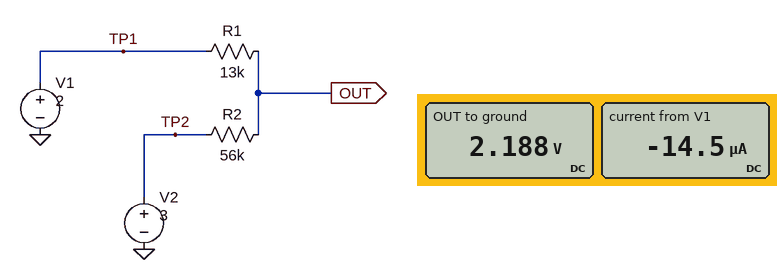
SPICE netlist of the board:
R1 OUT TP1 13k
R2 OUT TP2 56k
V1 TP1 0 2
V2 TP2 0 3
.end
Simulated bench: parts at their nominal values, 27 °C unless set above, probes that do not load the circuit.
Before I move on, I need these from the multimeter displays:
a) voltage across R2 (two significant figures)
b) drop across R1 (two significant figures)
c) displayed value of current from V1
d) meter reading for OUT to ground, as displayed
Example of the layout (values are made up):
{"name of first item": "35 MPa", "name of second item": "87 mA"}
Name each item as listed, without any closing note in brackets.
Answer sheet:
{"voltage across R2": "810 mV", "drop across R1": "190 mV", "displayed value of current from V1": "-14.5 µA", "meter reading for OUT to ground, as displayed": "2.188 V"}
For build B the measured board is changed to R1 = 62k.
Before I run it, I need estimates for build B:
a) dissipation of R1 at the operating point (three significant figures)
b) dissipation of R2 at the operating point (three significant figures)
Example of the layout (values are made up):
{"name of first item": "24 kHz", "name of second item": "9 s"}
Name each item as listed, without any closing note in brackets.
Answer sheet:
{"dissipation of R1 at the operating point": "4.45 µW", "dissipation of R2 at the operating point": "4.02 µW"}
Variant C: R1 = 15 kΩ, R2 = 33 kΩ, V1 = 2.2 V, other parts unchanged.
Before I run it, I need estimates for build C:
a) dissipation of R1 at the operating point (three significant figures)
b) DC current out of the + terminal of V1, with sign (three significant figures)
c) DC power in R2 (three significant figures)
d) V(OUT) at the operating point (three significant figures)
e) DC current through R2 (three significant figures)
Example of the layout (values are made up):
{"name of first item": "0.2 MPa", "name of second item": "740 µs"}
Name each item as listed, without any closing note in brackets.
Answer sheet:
{"dissipation of R1 at the operating point": "4.17 µW", "DC current out of the + terminal of V1, with sign": "-16.7 µA", "DC power in R2": "9.17 µW", "V(OUT) at the operating point": "2.45 V", "DC current through R2": "16.7 µA"}
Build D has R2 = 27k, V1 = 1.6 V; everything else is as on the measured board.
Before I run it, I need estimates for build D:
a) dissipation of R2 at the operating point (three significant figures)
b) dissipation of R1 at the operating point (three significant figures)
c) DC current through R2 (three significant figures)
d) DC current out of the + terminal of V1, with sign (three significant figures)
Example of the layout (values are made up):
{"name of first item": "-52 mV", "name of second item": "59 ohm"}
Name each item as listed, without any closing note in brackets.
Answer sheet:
{"dissipation of R2 at the operating point": "33.1 µW", "dissipation of R1 at the operating point": "15.9 µW", "DC current through R2": "35.0 µA", "DC current out of the + terminal of V1, with sign": "-35.0 µA"}
